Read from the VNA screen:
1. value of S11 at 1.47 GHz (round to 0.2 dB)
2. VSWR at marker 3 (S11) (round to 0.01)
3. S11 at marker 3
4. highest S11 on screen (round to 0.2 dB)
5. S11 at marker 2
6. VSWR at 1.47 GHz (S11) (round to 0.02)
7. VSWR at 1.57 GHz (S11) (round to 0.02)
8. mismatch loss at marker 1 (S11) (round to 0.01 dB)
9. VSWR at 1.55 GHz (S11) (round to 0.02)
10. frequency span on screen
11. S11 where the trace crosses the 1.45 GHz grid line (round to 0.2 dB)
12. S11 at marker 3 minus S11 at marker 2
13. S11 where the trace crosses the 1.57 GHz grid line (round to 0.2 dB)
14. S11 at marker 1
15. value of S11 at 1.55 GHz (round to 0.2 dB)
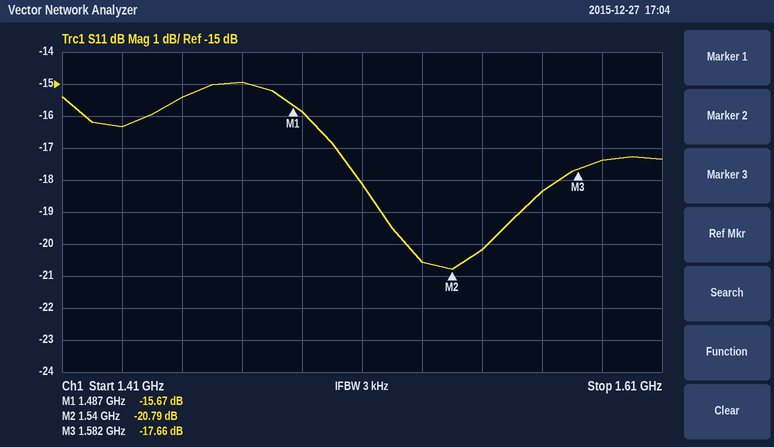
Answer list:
-15.0 dB
1.30
-17.66 dB
-15.0 dB
-20.79 dB
1.44
1.28
0.12 dB
1.22
200 MHz
-15.4 dB
3.13 dB
-18.4 dB
-15.67 dB
-20.2 dB
